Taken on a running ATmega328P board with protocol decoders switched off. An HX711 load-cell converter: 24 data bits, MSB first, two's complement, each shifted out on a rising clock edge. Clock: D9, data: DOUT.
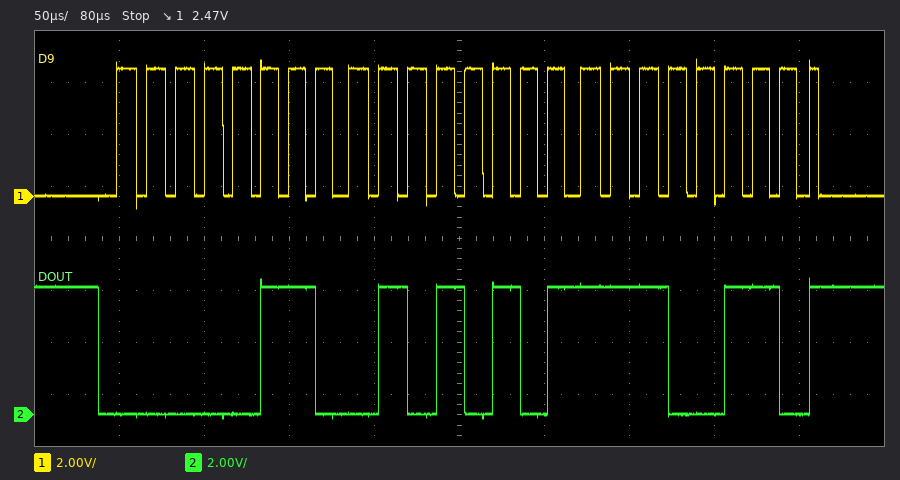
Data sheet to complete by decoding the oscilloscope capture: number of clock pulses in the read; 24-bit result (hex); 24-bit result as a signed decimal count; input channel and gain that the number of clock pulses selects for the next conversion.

25
0x0655E6
415206
channel A, gain 128
